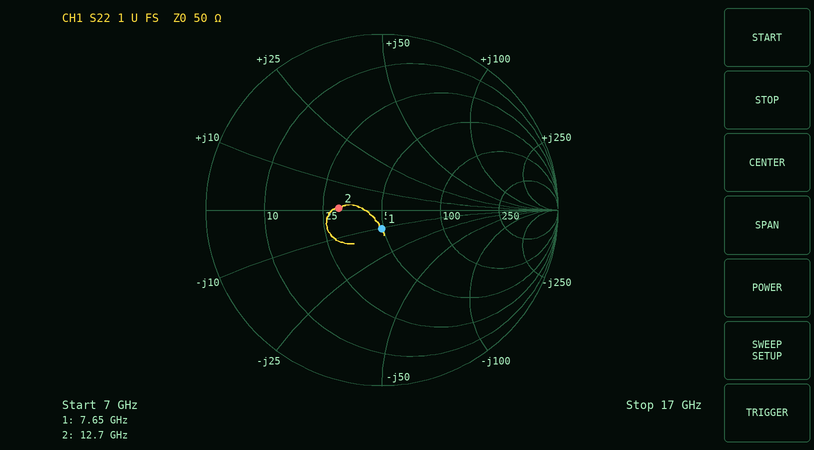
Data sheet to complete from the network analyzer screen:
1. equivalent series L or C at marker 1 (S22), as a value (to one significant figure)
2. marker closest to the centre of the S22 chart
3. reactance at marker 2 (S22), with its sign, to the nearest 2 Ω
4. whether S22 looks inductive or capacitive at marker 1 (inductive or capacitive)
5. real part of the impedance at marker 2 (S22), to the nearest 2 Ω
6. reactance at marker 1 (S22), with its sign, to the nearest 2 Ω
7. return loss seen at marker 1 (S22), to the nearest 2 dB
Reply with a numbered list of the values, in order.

1. 2 pF
2. marker 1
3. 0 Ω
4. capacitive
5. 30 Ω
6. -10 Ω
7. 20 dB
